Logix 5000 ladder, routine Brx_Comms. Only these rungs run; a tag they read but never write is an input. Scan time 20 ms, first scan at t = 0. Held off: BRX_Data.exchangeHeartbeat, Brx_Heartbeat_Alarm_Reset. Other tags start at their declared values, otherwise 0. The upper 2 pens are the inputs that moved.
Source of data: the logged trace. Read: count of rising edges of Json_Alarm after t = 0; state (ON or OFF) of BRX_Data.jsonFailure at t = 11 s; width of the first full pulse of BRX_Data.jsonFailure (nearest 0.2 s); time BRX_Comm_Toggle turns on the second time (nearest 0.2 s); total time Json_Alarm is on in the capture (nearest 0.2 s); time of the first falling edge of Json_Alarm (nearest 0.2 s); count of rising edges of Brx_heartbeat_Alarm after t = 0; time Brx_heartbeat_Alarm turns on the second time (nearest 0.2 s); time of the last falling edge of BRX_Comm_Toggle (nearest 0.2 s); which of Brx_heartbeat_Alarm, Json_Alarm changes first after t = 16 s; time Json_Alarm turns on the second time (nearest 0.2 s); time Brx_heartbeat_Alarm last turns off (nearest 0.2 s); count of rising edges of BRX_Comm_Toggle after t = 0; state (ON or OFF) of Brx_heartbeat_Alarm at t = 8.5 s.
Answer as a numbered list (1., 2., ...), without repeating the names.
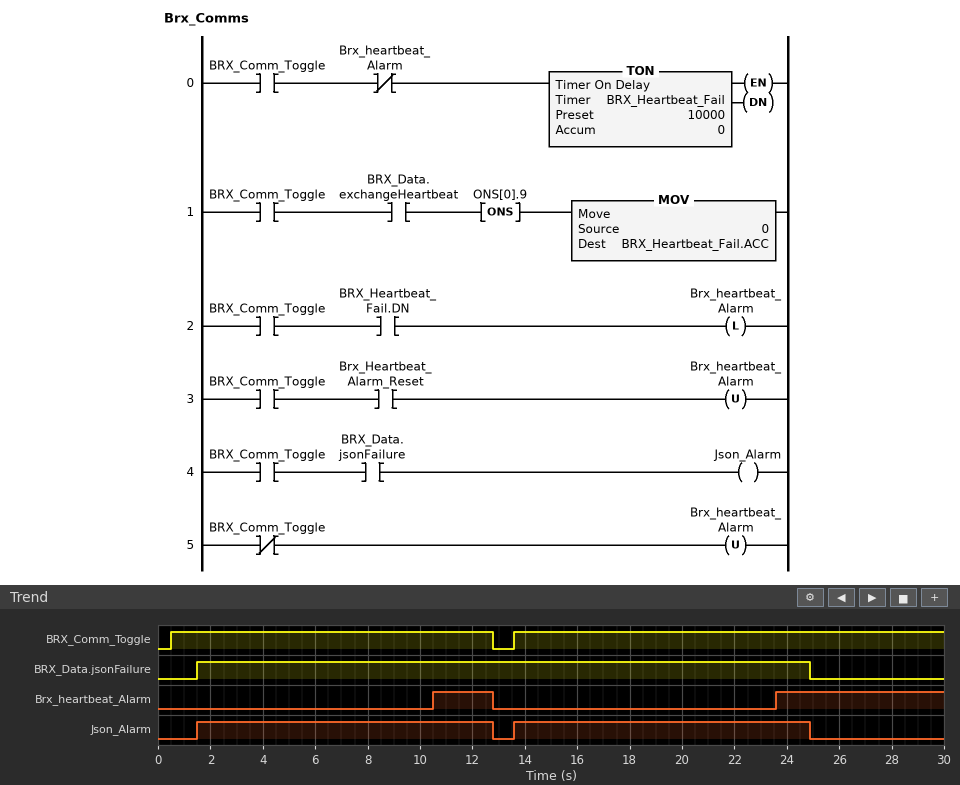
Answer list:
1. 2
2. ON
3. 23.4 s
4. 13.6 s
5. 22.6 s
6. 12.8 s
7. 2
8. 23.6 s
9. 12.8 s
10. Brx_heartbeat_Alarm
11. 13.6 s
12. 12.8 s
13. 2
14. OFF
